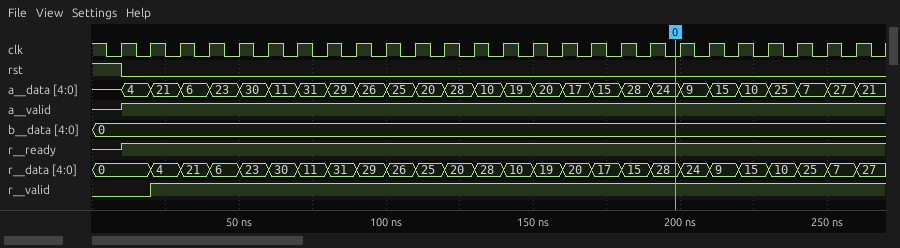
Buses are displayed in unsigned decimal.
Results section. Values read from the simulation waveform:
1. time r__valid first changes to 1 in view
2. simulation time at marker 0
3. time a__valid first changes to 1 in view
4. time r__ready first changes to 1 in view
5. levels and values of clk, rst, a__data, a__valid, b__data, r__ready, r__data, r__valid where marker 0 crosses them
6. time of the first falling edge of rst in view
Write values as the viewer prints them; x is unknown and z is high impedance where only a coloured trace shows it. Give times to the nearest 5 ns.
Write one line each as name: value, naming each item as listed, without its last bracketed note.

time r__valid first changes to 1 in view: 20 ns
simulation time at marker 0: 200 ns
time a__valid first changes to 1 in view: 10 ns
time r__ready first changes to 1 in view: 10 ns
levels and values of clk, rst, a__data, a__valid, b__data, r__ready, r__data, r__valid where marker 0 crosses them: clk=0, rst=0, a__data=24, a__valid=1, b__data=0, r__ready=1, r__data=28, r__valid=1
time of the first falling edge of rst in view: 10 ns
